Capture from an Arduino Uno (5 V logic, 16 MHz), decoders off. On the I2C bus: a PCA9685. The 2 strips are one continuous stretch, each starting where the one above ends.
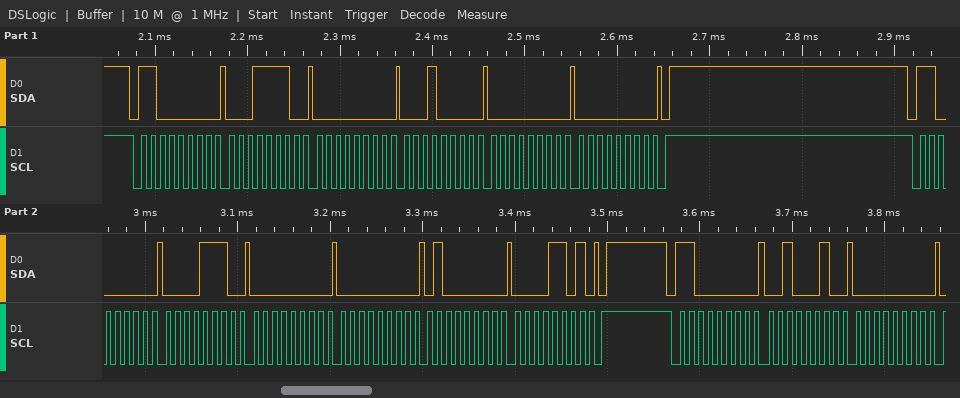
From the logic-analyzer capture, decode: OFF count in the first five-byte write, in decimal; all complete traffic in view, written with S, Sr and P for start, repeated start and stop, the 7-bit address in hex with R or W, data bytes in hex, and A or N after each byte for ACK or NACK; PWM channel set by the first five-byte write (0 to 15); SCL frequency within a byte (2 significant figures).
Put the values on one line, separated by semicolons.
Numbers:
0; S 60W A 1E A 00 A 10 A 00 A 00 A P S 60W A 0E A 00 A 00 A 40 A 0D A P S 60W A 22 A 00 A; 6; 100 kHz
